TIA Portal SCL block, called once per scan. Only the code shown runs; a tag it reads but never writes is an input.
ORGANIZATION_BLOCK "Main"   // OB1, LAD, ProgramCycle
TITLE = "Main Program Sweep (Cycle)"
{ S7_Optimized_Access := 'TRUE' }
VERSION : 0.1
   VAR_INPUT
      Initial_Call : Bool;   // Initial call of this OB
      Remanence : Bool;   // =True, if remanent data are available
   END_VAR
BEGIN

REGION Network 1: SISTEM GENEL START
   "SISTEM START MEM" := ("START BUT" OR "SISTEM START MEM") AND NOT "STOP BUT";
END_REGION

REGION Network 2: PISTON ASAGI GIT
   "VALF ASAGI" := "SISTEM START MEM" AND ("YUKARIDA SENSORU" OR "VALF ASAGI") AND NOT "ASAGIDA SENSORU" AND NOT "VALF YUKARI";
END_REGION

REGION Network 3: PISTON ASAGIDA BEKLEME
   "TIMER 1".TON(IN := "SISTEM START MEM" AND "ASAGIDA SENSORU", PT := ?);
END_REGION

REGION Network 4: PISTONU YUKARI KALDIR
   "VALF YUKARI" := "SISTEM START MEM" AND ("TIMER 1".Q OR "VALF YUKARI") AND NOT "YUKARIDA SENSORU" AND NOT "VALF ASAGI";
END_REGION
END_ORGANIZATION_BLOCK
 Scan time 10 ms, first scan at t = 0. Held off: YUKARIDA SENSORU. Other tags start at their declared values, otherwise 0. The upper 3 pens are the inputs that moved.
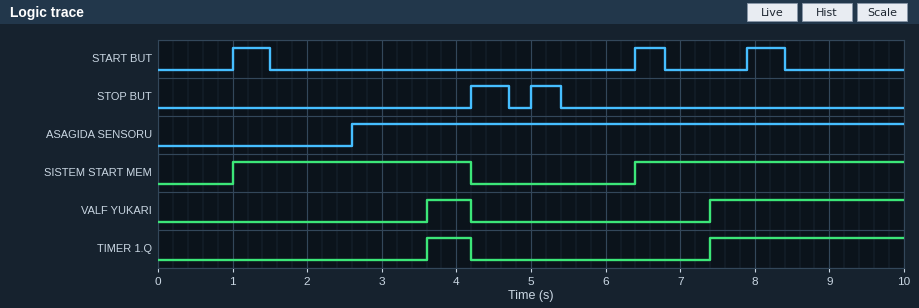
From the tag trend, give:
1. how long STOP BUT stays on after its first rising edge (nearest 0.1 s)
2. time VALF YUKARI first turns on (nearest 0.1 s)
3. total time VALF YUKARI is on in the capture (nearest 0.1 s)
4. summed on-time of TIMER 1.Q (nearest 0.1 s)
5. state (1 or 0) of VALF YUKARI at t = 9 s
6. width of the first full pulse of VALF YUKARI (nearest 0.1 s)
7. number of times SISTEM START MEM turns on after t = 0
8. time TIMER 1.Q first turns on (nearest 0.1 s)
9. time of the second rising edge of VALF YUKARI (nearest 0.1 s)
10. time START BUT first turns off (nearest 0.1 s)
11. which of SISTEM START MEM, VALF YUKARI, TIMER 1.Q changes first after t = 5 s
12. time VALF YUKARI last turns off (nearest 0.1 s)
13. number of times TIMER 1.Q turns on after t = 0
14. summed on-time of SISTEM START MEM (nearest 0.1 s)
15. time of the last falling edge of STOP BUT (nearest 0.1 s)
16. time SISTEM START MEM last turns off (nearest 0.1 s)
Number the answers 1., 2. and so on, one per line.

1. 0.5 s
2. 3.6 s
3. 3.2 s
4. 3.2 s
5. 1
6. 0.6 s
7. 2
8. 3.6 s
9. 7.4 s
10. 1.5 s
11. SISTEM START MEM
12. 4.2 s
13. 2
14. 6.8 s
15. 5.4 s
16. 4.2 s
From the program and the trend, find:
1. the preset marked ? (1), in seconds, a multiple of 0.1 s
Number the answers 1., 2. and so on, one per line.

1. 1.0 s
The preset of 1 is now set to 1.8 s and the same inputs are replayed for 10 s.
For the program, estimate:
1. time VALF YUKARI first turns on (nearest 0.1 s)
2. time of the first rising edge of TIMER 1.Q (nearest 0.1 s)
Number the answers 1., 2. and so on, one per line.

1. 8.2 s
2. 8.2 s
